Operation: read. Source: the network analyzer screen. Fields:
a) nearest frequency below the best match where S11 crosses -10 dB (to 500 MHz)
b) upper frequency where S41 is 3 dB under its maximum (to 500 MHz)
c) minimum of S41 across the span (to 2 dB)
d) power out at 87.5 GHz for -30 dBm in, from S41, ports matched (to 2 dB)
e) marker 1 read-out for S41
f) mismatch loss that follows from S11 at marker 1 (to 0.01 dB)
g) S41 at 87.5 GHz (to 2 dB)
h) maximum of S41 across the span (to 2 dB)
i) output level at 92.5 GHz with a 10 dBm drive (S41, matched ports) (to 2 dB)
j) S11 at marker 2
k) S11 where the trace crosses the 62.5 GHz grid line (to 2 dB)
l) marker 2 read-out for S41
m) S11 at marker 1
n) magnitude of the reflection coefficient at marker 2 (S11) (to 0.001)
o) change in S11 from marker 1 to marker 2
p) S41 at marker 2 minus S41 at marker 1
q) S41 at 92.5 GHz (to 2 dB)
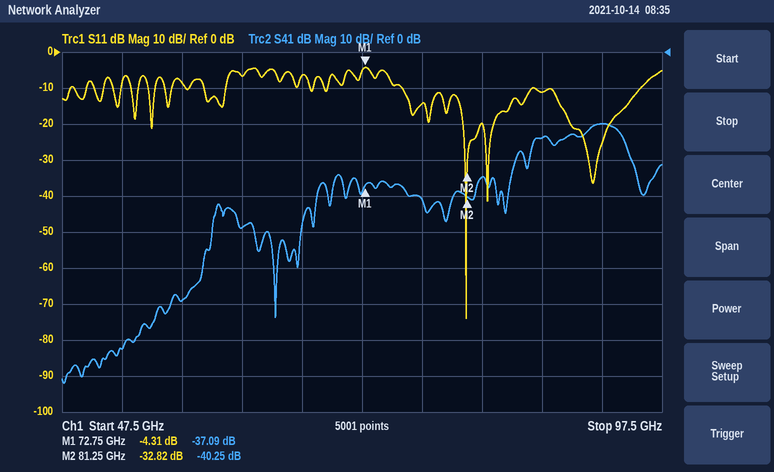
76.0 GHz
94.0 GHz
-92 dB
-54 dBm
-37.09 dB
2.01 dB
-24 dB
-20 dB
-10 dBm
-32.82 dB
-6 dB
-40.25 dB
-4.31 dB
0.023
-28.51 dB
-3.16 dB
-20 dB
